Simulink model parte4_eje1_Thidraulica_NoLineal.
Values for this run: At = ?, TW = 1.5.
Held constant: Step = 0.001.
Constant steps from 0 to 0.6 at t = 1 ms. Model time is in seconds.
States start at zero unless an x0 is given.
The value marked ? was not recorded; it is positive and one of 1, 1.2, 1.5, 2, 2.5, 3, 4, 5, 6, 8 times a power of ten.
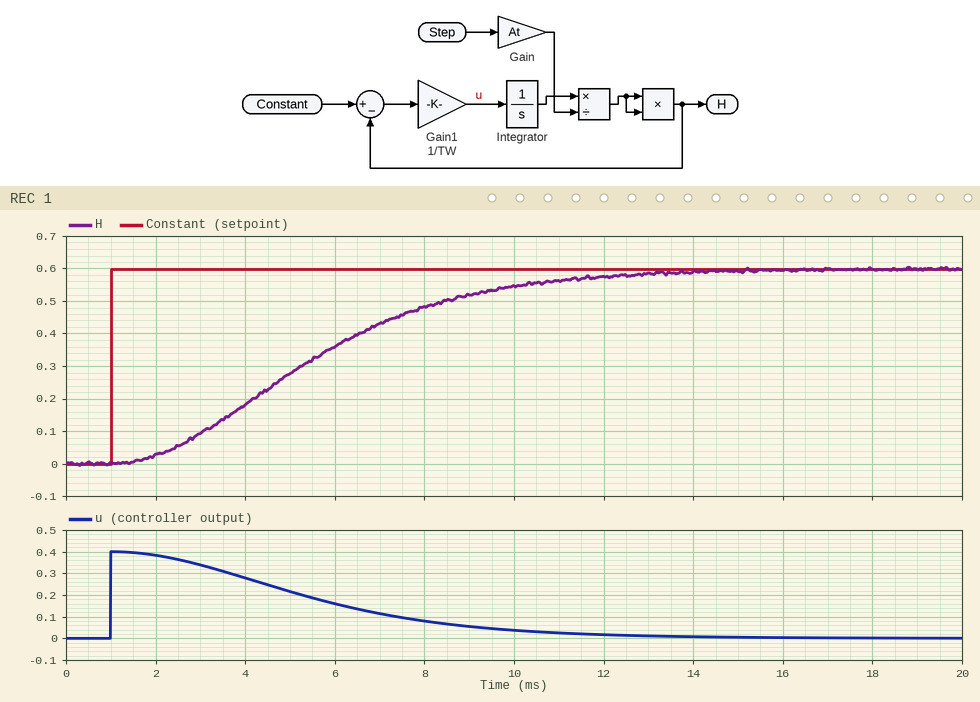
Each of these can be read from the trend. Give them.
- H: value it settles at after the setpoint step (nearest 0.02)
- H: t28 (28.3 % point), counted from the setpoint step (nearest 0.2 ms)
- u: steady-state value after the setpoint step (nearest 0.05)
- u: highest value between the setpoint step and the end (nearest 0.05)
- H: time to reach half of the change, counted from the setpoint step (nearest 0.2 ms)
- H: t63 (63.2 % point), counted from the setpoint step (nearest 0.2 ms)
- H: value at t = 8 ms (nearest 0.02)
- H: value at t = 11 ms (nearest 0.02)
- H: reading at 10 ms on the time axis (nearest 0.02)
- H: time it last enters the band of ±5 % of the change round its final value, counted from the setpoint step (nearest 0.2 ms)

0.60
2.8 ms
0.00
0.40
4.2 ms
5.2 ms
0.48
0.56
0.54
10.6 ms
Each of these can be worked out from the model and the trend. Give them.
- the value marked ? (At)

2.5
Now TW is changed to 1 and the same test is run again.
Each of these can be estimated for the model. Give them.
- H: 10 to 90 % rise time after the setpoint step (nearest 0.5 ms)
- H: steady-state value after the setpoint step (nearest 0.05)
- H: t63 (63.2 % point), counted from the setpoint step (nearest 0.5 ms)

5.0 ms
0.60
3.5 ms
